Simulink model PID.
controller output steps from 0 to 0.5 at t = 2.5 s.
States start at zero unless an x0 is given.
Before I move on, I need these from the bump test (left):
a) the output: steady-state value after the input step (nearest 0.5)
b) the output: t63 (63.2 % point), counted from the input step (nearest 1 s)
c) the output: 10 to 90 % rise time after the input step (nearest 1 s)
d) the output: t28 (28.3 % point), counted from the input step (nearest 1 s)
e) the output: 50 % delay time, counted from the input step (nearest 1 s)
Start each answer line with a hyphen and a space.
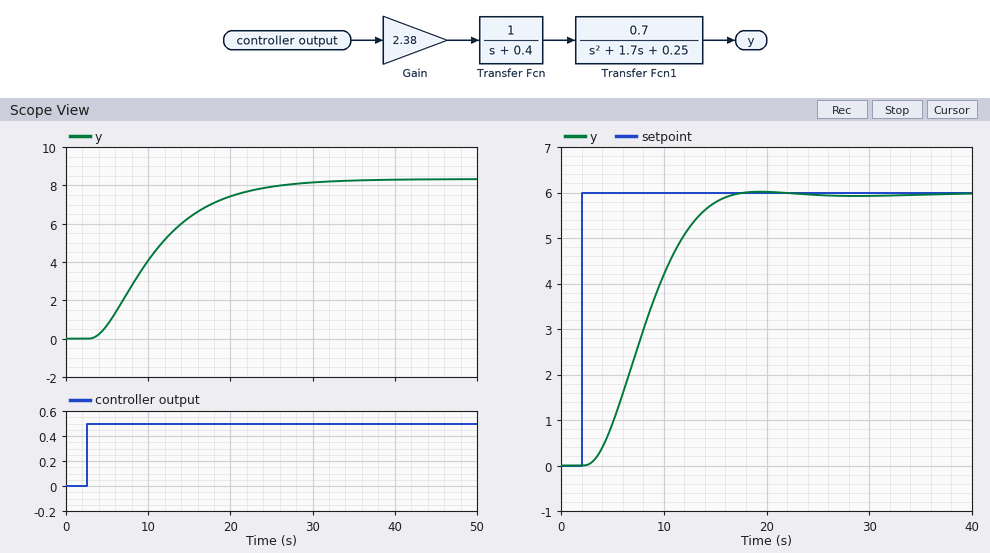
- 8.5
- 10 s
- 15 s
- 5 s
- 8 s
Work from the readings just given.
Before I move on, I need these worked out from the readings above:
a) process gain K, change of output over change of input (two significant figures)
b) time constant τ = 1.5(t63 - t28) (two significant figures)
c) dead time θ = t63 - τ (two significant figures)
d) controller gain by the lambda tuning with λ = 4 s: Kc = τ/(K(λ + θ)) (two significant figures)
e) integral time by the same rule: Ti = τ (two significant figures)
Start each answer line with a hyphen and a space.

- 17
- 7.5 s
- 2.5 s
- 0.068
- 7.5 s
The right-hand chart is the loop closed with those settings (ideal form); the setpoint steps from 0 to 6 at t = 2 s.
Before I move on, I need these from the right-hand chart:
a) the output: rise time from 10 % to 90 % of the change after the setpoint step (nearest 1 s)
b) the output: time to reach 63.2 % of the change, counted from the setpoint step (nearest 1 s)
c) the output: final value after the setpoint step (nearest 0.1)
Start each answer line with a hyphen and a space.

- 9 s
- 7 s
- 6.0
